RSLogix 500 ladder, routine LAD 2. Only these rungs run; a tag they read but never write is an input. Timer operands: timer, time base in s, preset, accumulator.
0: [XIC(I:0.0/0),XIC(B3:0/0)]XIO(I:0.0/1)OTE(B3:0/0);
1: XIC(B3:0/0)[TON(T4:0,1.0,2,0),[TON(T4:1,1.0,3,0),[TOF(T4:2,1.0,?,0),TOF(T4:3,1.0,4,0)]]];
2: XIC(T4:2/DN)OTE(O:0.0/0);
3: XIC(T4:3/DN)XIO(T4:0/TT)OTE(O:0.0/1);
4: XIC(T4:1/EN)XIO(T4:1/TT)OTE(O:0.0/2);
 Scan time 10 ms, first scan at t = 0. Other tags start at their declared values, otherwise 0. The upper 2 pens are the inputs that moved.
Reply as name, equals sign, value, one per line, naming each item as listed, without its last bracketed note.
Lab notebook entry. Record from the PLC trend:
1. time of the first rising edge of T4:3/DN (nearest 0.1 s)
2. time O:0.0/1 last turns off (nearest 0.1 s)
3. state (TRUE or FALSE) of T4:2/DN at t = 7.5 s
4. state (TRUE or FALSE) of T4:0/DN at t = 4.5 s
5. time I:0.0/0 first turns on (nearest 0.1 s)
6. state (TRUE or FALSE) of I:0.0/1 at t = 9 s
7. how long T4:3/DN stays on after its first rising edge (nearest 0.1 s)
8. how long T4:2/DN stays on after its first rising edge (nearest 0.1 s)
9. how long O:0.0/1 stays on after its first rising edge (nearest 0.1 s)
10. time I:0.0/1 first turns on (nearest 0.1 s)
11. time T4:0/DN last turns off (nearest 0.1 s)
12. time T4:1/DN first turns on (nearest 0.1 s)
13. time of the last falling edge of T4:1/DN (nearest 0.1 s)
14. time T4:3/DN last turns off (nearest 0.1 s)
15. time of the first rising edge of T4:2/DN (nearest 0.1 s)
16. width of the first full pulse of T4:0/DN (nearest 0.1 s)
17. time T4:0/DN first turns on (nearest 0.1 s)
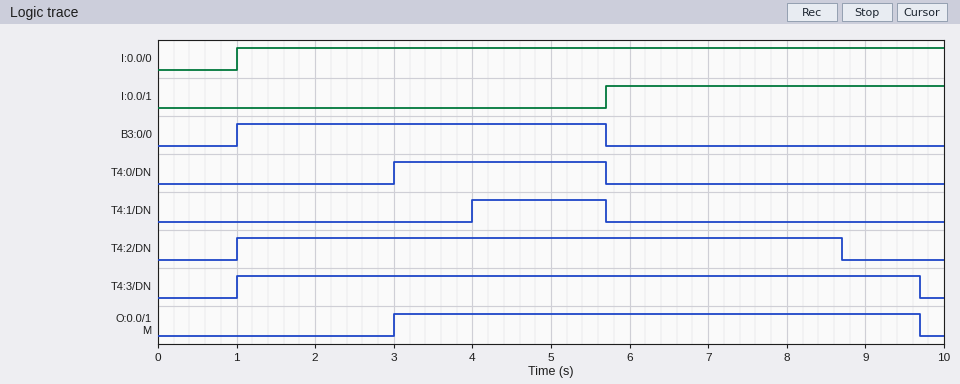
time of the first rising edge of T4:3/DN = 1.0 s
time O:0.0/1 last turns off = 9.7 s
state (TRUE or FALSE) of T4:2/DN at t = 7.5 s = TRUE
state (TRUE or FALSE) of T4:0/DN at t = 4.5 s = TRUE
time I:0.0/0 first turns on = 1.0 s
state (TRUE or FALSE) of I:0.0/1 at t = 9 s = TRUE
how long T4:3/DN stays on after its first rising edge = 8.7 s
how long T4:2/DN stays on after its first rising edge = 7.7 s
how long O:0.0/1 stays on after its first rising edge = 6.7 s
time I:0.0/1 first turns on = 5.7 s
time T4:0/DN last turns off = 5.7 s
time T4:1/DN first turns on = 4.0 s
time of the last falling edge of T4:1/DN = 5.7 s
time T4:3/DN last turns off = 9.7 s
time of the first rising edge of T4:2/DN = 1.0 s
width of the first full pulse of T4:0/DN = 2.7 s
time T4:0/DN first turns on = 3.0 s
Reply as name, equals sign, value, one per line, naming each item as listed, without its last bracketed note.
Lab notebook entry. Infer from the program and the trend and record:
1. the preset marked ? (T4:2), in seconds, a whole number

the preset marked ? (T4:2), in seconds, a whole number = 3 s
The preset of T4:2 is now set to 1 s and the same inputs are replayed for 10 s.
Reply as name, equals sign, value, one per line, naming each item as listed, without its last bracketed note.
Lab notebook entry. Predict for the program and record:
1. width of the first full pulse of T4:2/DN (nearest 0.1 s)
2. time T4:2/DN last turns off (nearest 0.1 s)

width of the first full pulse of T4:2/DN = 5.7 s
time T4:2/DN last turns off = 6.7 s
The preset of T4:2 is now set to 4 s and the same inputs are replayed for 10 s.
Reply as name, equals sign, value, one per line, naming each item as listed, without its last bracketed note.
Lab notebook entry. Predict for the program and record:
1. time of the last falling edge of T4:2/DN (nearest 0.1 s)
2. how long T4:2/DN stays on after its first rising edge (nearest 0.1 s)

time of the last falling edge of T4:2/DN = 9.7 s
how long T4:2/DN stays on after its first rising edge = 8.7 s
